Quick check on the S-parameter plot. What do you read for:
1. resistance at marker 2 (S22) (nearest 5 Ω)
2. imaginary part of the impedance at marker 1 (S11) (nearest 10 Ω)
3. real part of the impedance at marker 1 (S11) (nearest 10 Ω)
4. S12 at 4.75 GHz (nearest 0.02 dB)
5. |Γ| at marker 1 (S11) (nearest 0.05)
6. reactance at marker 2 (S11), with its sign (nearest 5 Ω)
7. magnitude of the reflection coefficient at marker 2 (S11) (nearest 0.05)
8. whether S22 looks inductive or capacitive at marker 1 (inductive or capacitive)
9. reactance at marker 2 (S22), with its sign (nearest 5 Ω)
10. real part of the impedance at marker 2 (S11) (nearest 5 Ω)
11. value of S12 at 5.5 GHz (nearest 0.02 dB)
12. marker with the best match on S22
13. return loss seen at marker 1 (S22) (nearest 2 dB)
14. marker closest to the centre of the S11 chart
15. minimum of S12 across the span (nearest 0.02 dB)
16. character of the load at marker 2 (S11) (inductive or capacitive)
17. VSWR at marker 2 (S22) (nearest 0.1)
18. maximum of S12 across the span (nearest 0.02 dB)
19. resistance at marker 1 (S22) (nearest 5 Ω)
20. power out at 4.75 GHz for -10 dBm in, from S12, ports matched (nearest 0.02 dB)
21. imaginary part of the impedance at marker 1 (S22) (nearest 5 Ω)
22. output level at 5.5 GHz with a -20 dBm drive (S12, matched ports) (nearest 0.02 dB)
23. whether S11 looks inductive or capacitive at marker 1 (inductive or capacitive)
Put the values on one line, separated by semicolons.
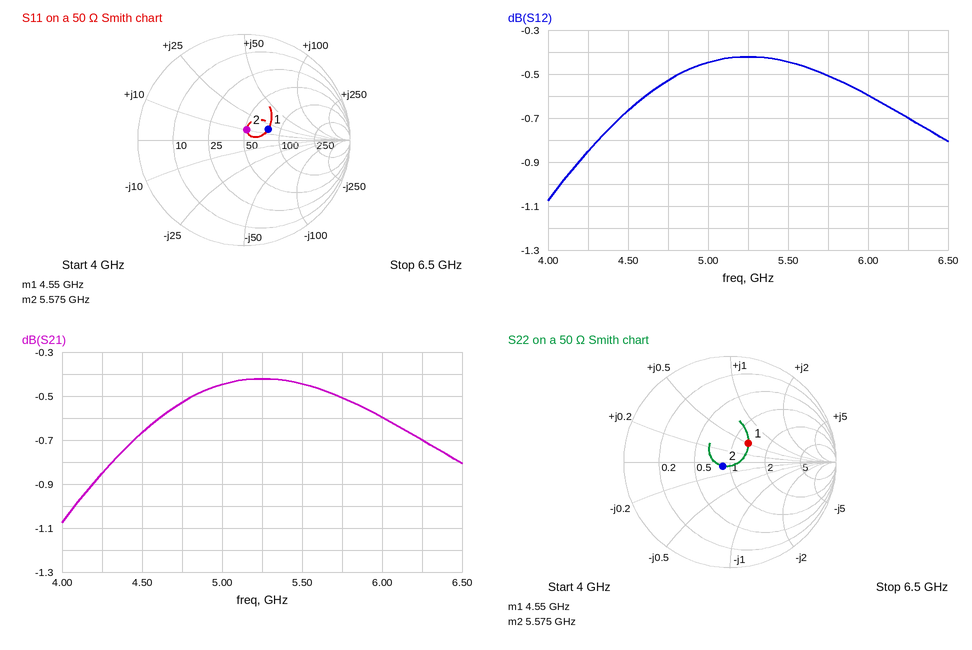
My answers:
45 Ω; +20 Ω; 80 Ω; -0.52 dB; 0.25; +10 Ω; 0.10; inductive; -5 Ω; 50 Ω; -0.44 dB; marker 2; 12 dB; marker 2; -1.08 dB; inductive; 1.2; -0.42 dB; 65 Ω; -10.52 dBm; +25 Ω; -20.44 dBm; inductive
